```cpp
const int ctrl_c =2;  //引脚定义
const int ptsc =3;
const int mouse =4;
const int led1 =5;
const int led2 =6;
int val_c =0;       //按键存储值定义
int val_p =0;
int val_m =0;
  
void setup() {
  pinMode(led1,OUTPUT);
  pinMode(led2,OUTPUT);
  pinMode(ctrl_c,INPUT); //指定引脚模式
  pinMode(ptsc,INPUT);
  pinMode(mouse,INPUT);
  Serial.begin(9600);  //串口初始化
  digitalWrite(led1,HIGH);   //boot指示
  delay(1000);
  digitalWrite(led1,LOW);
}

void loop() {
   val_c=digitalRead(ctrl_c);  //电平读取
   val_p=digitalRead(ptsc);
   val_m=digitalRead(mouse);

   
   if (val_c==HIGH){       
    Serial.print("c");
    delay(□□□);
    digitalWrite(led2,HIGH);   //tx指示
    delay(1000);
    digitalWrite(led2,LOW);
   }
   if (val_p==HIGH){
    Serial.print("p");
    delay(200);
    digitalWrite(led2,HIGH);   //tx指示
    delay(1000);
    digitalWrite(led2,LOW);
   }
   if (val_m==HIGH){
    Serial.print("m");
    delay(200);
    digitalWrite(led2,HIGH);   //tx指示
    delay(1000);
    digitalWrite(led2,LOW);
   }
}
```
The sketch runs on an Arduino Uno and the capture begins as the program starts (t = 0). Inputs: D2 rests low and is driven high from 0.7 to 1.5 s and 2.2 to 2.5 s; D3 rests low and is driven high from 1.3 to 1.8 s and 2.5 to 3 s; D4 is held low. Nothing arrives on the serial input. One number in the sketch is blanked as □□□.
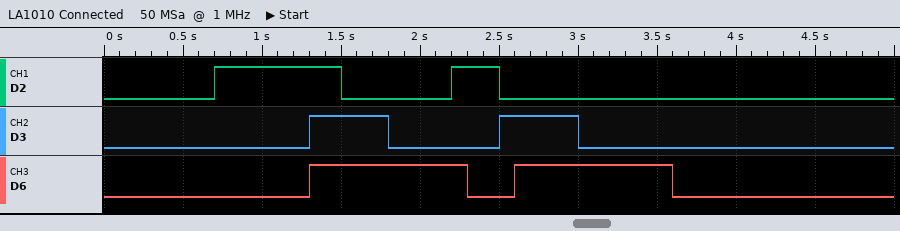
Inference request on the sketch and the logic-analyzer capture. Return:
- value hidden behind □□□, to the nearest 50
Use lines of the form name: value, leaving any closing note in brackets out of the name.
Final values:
value hidden behind □□□, to the nearest 50: 300
